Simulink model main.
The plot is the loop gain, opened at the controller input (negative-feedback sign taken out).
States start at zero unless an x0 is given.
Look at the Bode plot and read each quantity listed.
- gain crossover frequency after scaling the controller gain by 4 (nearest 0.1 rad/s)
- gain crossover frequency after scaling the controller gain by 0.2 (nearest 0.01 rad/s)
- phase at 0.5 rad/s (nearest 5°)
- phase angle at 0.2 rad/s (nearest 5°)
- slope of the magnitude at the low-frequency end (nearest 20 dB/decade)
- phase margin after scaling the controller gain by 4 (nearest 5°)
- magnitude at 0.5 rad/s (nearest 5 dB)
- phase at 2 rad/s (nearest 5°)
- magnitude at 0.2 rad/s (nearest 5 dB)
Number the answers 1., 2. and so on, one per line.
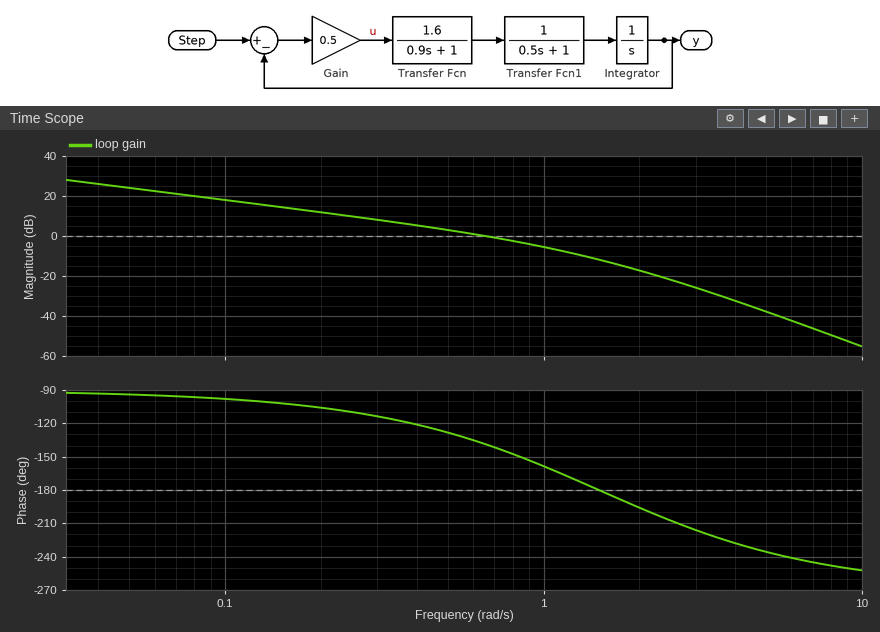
1. 1.5 rad/s
2. 0.16 rad/s
3. -130°
4. -105°
5. -20 dB/decade
6. 0°
7. 5 dB
8. -195°
9. 10 dB
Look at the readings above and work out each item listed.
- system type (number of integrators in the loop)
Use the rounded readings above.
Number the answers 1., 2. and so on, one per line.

1. 1
